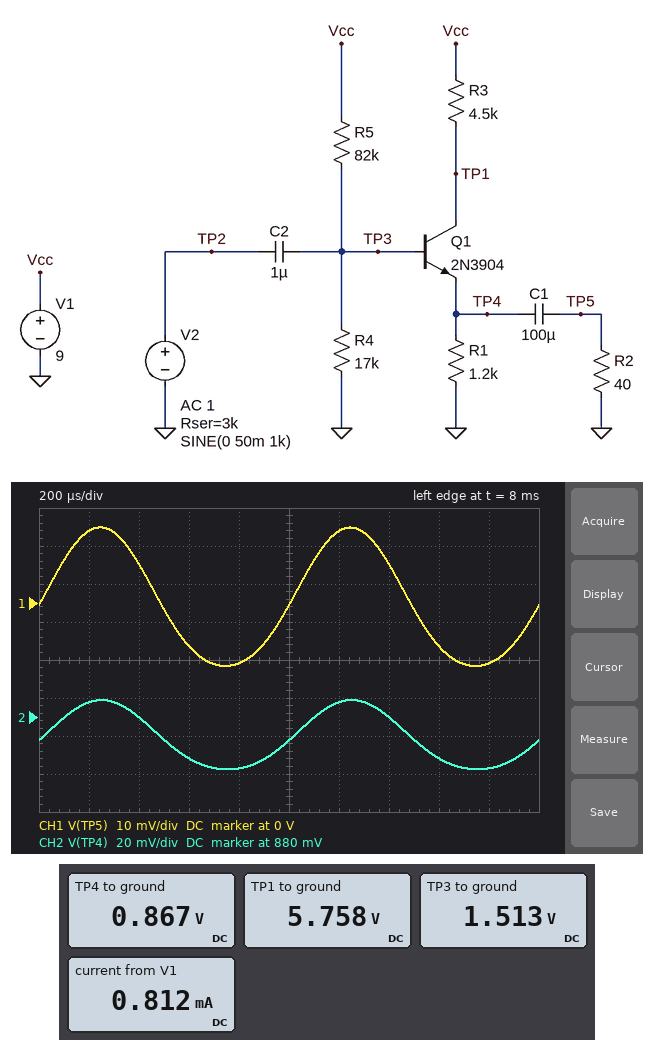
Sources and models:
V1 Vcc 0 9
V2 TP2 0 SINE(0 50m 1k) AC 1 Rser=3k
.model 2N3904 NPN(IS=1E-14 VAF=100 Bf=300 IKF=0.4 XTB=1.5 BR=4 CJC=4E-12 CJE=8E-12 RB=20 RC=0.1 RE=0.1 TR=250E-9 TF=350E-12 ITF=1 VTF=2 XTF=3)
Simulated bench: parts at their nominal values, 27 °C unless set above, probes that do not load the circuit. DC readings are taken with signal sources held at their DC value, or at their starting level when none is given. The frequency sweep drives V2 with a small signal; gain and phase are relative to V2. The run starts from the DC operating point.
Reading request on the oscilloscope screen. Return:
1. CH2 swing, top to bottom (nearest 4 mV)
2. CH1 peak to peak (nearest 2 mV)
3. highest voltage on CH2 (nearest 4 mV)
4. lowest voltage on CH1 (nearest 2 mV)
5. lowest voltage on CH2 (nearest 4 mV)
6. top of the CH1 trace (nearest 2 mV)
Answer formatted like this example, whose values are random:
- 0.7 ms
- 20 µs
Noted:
- 36 mV
- 36 mV
- 888 mV
- -16 mV
- 852 mV
- 20 mV
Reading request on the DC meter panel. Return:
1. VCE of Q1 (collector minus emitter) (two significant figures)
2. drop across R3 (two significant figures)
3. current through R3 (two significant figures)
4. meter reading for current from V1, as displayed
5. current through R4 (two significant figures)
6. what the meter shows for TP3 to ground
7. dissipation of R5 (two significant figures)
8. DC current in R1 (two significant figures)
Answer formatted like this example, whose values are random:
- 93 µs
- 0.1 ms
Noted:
- 4.9 V
- 3.2 V
- 720 µA
- 0.812 mA
- 89 µA
- 1.513 V
- 680 µW
- 720 µA
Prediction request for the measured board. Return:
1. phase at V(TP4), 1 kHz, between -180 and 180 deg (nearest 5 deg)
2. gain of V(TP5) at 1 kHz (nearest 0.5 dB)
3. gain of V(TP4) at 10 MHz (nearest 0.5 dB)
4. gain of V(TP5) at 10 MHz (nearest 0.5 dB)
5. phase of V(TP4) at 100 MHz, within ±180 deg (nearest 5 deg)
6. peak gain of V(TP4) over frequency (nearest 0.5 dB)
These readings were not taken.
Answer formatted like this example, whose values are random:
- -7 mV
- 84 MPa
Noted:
- 0 deg
- -8.5 dB
- -33.0 dB
- -33.0 dB
- -5 deg
- -6.0 dB
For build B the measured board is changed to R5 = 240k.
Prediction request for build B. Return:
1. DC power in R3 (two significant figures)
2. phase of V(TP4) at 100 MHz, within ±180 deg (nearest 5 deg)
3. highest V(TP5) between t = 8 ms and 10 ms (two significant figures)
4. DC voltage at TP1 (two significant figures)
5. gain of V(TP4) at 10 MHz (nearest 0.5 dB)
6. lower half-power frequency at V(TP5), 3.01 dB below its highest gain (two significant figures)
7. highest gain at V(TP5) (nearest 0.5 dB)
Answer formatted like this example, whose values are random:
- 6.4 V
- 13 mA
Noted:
- 3.5 µW
- 5 deg
- 3.3 mV
- 8.9 V
- -38.5 dB
- 9.6 Hz
- -29.5 dB
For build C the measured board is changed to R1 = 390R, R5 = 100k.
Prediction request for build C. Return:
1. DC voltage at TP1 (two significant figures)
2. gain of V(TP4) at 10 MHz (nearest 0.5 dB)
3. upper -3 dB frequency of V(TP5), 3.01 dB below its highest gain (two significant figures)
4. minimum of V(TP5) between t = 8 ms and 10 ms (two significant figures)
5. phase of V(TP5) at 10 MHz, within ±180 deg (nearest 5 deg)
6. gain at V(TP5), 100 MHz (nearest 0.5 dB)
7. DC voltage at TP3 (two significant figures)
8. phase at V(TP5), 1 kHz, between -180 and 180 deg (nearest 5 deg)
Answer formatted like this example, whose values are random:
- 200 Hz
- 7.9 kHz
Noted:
- 2.4 V
- -35.0 dB
- 290 kHz
- -22 mV
- -50 deg
- -39.0 dB
- 1.2 V
- 0 deg
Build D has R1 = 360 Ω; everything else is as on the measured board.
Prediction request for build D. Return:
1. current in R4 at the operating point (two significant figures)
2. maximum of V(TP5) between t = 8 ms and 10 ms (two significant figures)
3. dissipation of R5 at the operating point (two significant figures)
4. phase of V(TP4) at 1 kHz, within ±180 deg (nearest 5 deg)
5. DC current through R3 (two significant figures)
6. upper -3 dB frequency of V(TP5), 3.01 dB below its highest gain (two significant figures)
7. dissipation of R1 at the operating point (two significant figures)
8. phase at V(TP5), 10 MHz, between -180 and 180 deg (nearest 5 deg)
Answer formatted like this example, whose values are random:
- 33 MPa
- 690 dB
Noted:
- 79 µA
- 1.3 mV
- 720 µW
- 0 deg
- 1.8 mA
- 360 kHz
- 1.2 mW
- 0 deg
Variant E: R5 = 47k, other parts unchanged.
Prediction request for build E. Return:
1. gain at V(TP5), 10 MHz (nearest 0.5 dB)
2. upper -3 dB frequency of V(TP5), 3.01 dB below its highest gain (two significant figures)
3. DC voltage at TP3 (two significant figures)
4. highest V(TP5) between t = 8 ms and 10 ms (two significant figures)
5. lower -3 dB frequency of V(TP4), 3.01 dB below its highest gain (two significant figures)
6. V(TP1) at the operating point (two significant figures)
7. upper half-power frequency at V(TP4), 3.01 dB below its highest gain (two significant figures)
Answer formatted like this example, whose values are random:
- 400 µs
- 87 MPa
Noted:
- -35.5 dB
- 260 kHz
- 2.3 V
- 9.2 mV
- 6.4 Hz
- 2.8 V
- 200 kHz
